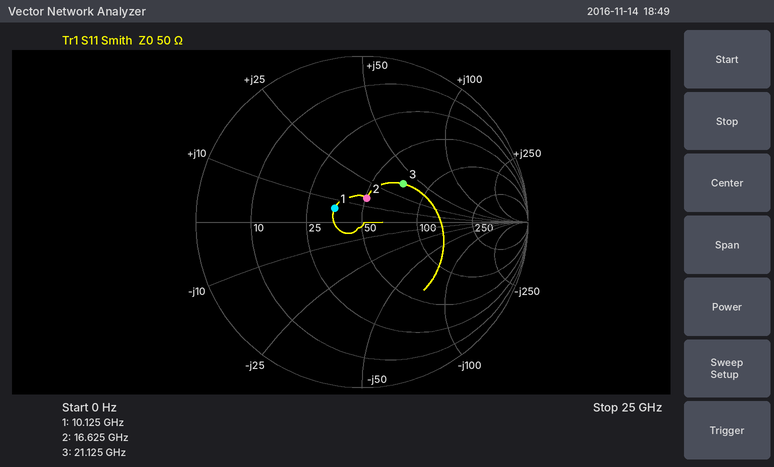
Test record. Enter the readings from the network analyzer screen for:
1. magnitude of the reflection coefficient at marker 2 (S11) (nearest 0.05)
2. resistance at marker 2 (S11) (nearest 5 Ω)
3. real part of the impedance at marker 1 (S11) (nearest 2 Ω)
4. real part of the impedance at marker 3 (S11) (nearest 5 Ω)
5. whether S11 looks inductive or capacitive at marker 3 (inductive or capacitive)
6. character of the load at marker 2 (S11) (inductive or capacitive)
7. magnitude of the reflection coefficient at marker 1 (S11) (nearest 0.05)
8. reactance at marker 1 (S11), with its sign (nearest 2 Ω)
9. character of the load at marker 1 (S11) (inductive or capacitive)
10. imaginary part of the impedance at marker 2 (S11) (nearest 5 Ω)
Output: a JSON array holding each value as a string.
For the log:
["0.15", "50 Ω", "36 Ω", "70 Ω", "inductive", "inductive", "0.20", "+6 Ω", "inductive", "+15 Ω"]
